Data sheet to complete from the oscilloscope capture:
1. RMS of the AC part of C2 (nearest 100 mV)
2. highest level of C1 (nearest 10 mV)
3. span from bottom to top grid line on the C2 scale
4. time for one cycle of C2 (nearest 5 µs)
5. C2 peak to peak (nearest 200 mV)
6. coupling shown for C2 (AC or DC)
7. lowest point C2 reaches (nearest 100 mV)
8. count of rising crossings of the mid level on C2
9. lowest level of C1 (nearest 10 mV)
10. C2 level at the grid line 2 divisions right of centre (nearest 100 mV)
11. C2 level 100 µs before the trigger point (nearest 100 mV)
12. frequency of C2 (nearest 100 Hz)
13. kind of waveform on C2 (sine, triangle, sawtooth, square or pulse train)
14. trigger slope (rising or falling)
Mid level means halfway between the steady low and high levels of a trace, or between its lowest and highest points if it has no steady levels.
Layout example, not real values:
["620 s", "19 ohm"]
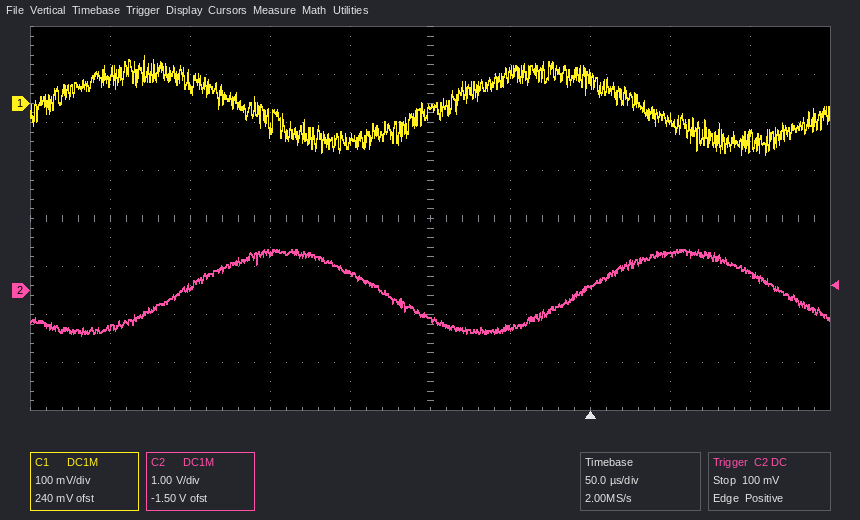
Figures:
["600 mV", "100 mV", "8 V", "250 µs", "1.8 V", "DC", "-900 mV", "2", "-110 mV", "100 mV", "-600 mV", "4.0 kHz", "sine", "rising"]
